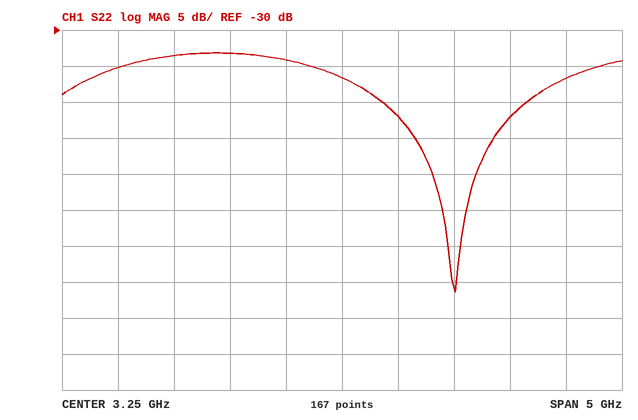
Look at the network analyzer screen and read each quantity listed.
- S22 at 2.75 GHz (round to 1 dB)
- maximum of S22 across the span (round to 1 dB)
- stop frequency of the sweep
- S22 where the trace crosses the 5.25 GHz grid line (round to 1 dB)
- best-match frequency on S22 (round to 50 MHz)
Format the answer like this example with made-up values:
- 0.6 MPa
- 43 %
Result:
- -34 dB
- -33 dB
- 5.75 GHz
- -37 dB
- 4.25 GHz
